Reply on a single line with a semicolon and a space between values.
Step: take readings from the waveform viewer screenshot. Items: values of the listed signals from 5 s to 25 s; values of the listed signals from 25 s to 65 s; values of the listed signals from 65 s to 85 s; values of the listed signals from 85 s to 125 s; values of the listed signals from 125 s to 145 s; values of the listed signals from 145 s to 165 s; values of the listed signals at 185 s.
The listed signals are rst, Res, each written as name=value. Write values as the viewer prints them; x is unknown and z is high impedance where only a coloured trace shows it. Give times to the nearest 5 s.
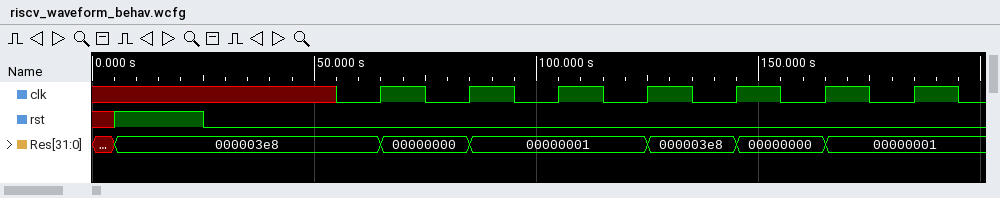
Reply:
rst=1, Res=000003e8; rst=0, Res=000003e8; rst=0, Res=00000000; rst=0, Res=00000001; rst=0, Res=000003e8; rst=0, Res=00000000; rst=0, Res=00000001
